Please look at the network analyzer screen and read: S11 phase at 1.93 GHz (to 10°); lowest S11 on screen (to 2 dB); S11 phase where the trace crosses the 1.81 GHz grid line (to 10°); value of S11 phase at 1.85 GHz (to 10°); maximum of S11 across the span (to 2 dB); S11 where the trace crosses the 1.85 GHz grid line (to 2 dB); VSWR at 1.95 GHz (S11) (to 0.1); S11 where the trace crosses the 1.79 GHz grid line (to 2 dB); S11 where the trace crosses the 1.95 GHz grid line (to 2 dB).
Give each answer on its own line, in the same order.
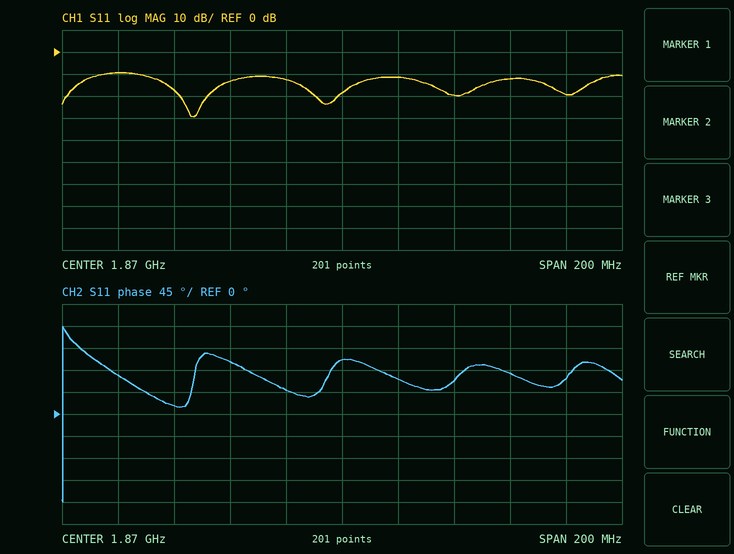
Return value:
80°
-30 dB
20°
50°
-10 dB
-12 dB
1.2
-10 dB
-20 dB
